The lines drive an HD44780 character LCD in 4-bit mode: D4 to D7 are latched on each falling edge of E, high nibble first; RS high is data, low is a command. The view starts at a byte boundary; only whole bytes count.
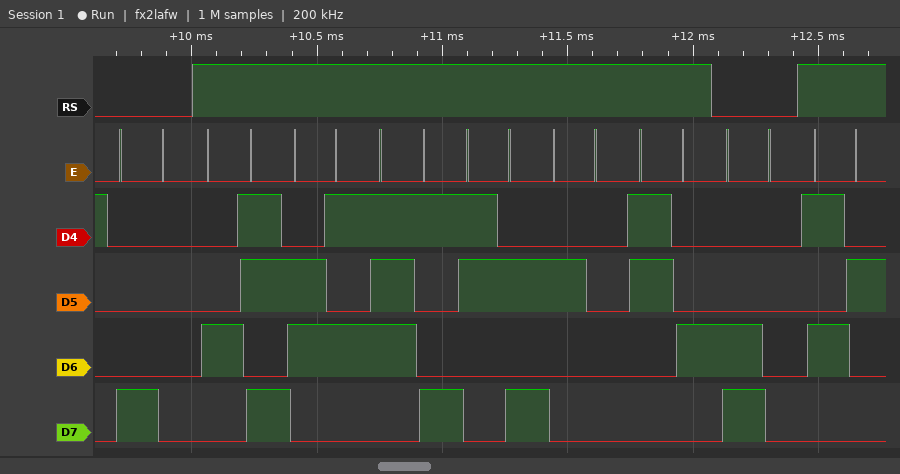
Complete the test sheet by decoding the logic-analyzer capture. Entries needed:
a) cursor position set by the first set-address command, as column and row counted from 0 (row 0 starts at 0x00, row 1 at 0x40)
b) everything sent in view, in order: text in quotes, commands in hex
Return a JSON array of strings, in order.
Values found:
["column 0, row 0", "0x80 \"Key: 4\" 0xC0 \"R\""]
